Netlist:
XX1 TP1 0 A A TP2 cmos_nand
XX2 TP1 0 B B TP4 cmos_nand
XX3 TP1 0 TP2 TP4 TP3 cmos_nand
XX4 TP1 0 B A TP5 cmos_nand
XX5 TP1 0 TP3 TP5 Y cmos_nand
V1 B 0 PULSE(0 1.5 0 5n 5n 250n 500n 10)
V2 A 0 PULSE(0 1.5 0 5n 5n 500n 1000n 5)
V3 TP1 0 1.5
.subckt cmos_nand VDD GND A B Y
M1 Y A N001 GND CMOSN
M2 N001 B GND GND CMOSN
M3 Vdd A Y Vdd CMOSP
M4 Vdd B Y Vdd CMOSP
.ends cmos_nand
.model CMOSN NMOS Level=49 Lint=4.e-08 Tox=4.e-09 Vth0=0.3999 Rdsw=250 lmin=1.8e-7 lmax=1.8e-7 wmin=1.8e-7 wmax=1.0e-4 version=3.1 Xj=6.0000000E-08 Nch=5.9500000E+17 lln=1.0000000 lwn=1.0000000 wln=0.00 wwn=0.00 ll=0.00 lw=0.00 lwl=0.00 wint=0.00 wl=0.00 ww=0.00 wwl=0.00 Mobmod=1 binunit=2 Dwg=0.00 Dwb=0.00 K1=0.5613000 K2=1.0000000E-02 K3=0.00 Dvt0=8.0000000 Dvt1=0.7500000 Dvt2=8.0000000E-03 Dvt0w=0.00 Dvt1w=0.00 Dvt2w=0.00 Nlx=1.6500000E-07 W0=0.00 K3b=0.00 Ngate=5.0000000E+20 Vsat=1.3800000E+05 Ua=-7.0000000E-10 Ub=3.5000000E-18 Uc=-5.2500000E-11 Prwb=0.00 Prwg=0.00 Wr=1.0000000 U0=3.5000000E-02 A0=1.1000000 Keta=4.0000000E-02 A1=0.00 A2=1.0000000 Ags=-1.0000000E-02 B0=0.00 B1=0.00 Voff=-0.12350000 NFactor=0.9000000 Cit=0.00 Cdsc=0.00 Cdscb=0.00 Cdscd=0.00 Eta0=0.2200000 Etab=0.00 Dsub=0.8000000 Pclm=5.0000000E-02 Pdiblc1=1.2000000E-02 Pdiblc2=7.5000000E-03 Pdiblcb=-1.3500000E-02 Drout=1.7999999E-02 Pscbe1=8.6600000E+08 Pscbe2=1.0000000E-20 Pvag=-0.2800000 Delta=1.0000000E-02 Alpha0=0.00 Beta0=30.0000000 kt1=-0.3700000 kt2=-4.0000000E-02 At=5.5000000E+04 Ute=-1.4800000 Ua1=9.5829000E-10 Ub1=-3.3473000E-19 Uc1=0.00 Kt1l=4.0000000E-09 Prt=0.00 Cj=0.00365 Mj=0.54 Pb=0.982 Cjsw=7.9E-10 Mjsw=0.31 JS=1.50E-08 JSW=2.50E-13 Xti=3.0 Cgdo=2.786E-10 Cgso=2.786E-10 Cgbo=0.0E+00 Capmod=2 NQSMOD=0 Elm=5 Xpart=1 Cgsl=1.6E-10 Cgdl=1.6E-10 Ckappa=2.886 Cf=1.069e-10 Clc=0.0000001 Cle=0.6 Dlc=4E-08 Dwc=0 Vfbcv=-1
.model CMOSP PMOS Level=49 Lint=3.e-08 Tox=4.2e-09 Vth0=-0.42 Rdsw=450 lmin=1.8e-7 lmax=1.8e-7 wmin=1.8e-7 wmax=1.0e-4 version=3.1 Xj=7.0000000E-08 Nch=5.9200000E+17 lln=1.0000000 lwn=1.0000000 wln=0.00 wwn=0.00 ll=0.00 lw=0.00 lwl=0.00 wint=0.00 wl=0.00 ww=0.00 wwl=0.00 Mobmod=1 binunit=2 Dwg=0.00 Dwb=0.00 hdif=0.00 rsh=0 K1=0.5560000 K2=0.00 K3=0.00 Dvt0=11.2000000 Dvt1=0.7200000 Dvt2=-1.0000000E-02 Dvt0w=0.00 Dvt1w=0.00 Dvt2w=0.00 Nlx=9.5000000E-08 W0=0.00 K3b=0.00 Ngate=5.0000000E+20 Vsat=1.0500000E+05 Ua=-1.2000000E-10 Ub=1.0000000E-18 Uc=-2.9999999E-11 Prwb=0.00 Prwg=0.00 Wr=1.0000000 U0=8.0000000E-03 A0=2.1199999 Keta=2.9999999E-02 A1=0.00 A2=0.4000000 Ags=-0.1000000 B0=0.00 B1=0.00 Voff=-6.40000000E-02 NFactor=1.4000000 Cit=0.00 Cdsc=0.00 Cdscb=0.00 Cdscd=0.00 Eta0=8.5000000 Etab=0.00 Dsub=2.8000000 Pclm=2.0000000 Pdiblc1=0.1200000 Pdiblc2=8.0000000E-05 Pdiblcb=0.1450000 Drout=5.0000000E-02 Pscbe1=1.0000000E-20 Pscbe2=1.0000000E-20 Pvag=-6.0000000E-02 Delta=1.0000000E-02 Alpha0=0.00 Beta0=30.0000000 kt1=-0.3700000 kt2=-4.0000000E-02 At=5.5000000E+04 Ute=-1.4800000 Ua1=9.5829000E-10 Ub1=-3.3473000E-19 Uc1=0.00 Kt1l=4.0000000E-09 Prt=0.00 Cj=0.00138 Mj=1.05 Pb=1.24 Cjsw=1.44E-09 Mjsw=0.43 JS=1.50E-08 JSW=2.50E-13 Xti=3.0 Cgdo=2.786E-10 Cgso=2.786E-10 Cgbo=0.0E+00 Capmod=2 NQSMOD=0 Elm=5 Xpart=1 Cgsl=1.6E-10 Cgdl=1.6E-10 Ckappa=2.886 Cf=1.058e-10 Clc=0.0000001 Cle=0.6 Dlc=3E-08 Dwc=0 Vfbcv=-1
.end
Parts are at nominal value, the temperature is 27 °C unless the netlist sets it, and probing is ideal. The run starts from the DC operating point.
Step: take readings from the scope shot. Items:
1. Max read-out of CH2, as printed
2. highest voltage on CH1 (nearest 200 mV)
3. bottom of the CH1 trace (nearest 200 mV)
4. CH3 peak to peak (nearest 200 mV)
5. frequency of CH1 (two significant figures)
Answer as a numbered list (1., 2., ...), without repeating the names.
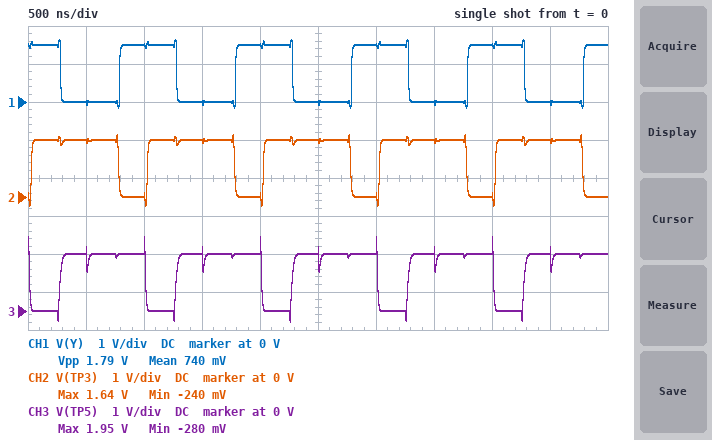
1. 1.64 V
2. 1.6 V
3. -200 mV
4. 2.2 V
5. 1.0 MHz
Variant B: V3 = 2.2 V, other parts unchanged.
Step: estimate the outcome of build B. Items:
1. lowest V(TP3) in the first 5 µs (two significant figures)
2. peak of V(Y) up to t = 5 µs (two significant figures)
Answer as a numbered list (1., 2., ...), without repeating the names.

1. -170 mV
2. 2.4 V
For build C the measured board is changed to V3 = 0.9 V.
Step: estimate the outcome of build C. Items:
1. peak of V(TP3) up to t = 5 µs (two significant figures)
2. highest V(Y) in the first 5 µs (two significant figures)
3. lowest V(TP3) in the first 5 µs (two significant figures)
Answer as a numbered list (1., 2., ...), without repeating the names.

1. 1.0 V
2. 1.1 V
3. -260 mV
